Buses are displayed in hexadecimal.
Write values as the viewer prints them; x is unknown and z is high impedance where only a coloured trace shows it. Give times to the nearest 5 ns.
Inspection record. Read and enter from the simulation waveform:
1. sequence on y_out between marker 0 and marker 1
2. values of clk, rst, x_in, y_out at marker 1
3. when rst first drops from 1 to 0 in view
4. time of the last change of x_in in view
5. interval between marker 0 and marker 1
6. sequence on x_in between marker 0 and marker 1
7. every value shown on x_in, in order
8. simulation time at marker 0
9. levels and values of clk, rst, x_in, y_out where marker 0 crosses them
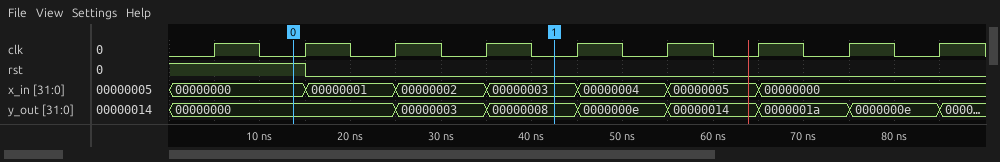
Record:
00000000, 00000003, 00000008
clk=0, rst=0, x_in=00000003, y_out=00000008
15 ns
65 ns
30 ns
00000000, 00000001, 00000002, 00000003
00000000, 00000001, 00000002, 00000003, 00000004, 00000005, 00000000
15 ns
clk=0, rst=1, x_in=00000000, y_out=00000000
